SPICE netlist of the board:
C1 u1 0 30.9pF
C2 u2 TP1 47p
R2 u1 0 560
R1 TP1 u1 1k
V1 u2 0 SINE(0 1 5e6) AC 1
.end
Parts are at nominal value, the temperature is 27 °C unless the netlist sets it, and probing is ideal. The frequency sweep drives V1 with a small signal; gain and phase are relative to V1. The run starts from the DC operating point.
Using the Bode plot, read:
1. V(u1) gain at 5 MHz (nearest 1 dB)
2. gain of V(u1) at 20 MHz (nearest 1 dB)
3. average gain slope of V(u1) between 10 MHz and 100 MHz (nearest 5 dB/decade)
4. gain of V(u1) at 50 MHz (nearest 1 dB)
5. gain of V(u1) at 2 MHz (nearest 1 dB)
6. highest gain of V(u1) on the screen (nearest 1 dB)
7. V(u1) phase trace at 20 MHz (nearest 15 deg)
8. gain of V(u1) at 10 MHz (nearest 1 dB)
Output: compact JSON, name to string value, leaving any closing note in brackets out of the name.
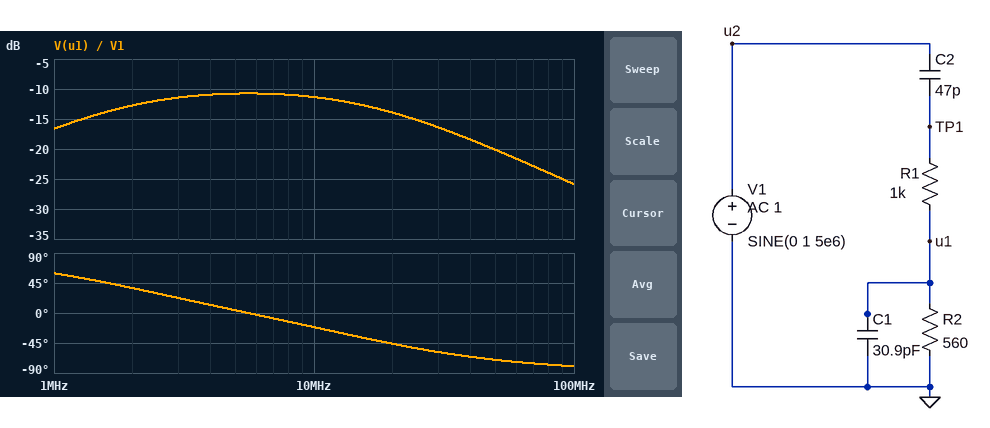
{"V(u1) gain at 5 MHz": "-11 dB", "gain of V(u1) at 20 MHz": "-14 dB", "average gain slope of V(u1) between 10 MHz and 100 MHz": "-15 dB/decade", "gain of V(u1) at 50 MHz": "-20 dB", "gain of V(u1) at 2 MHz": "-13 dB", "highest gain of V(u1) on the screen": "-11 dB", "V(u1) phase trace at 20 MHz": "-45 deg", "gain of V(u1) at 10 MHz": "-11 dB"}
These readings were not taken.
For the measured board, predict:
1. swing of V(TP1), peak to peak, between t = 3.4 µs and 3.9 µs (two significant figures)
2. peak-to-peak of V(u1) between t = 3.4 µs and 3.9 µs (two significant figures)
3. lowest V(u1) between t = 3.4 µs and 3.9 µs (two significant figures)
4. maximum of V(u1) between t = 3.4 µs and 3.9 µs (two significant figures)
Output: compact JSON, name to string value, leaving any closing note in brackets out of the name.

{"swing of V(TP1), peak to peak, between t = 3.4 µs and 3.9 µs": "1.7 V", "peak-to-peak of V(u1) between t = 3.4 µs and 3.9 µs": "580 mV", "lowest V(u1) between t = 3.4 µs and 3.9 µs": "-290 mV", "maximum of V(u1) between t = 3.4 µs and 3.9 µs": "290 mV"}
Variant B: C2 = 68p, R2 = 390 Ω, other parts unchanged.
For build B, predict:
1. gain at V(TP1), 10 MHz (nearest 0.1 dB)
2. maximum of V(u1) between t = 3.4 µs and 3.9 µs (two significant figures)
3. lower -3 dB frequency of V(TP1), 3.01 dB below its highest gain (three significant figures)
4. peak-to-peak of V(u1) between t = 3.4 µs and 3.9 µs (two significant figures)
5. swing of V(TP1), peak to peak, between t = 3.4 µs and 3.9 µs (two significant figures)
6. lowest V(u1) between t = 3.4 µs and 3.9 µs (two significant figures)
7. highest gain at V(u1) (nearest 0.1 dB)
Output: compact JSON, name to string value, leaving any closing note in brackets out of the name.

{"gain at V(TP1), 10 MHz": "-0.4 dB", "maximum of V(u1) between t = 3.4 µs and 3.9 µs": "250 mV", "lower -3 dB frequency of V(TP1), 3.01 dB below its highest gain": "1.75 MHz", "peak-to-peak of V(u1) between t = 3.4 µs and 3.9 µs": "500 mV", "swing of V(TP1), peak to peak, between t = 3.4 µs and 3.9 µs": "1.8 V", "lowest V(u1) between t = 3.4 µs and 3.9 µs": "-250 mV", "highest gain at V(u1)": "-12.1 dB"}
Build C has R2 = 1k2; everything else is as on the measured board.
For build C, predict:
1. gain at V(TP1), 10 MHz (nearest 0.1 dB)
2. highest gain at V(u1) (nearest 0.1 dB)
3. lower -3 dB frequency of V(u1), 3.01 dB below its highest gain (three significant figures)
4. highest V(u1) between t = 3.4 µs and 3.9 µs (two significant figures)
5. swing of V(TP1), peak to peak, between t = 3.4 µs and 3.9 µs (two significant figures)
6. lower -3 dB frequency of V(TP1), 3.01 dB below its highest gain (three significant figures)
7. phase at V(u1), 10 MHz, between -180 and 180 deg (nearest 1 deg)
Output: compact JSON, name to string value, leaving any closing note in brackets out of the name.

{"gain at V(TP1), 10 MHz": "-1.0 dB", "highest gain at V(u1)": "-7.9 dB", "lower -3 dB frequency of V(u1), 3.01 dB below its highest gain": "1.05 MHz", "highest V(u1) between t = 3.4 µs and 3.9 µs": "400 mV", "swing of V(TP1), peak to peak, between t = 3.4 µs and 3.9 µs": "1.6 V", "lower -3 dB frequency of V(TP1), 3.01 dB below its highest gain": "2.11 MHz", "phase at V(u1), 10 MHz, between -180 and 180 deg": "-34 deg"}
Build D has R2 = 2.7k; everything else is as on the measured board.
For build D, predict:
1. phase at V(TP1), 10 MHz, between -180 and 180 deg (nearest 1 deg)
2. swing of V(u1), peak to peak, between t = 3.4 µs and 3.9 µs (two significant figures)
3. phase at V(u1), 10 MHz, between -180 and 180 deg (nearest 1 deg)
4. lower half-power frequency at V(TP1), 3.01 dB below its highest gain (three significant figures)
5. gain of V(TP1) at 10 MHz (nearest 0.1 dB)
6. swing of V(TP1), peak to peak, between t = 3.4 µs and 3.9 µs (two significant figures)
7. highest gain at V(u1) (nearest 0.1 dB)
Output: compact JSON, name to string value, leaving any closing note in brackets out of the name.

{"phase at V(TP1), 10 MHz, between -180 and 180 deg": "13 deg", "swing of V(u1), peak to peak, between t = 3.4 µs and 3.9 µs": "930 mV", "phase at V(u1), 10 MHz, between -180 and 180 deg": "-42 deg", "lower half-power frequency at V(TP1), 3.01 dB below its highest gain": "2.23 MHz", "gain of V(TP1) at 10 MHz": "-1.2 dB", "swing of V(TP1), peak to peak, between t = 3.4 µs and 3.9 µs": "1.6 V", "highest gain at V(u1)": "-6.1 dB"}
